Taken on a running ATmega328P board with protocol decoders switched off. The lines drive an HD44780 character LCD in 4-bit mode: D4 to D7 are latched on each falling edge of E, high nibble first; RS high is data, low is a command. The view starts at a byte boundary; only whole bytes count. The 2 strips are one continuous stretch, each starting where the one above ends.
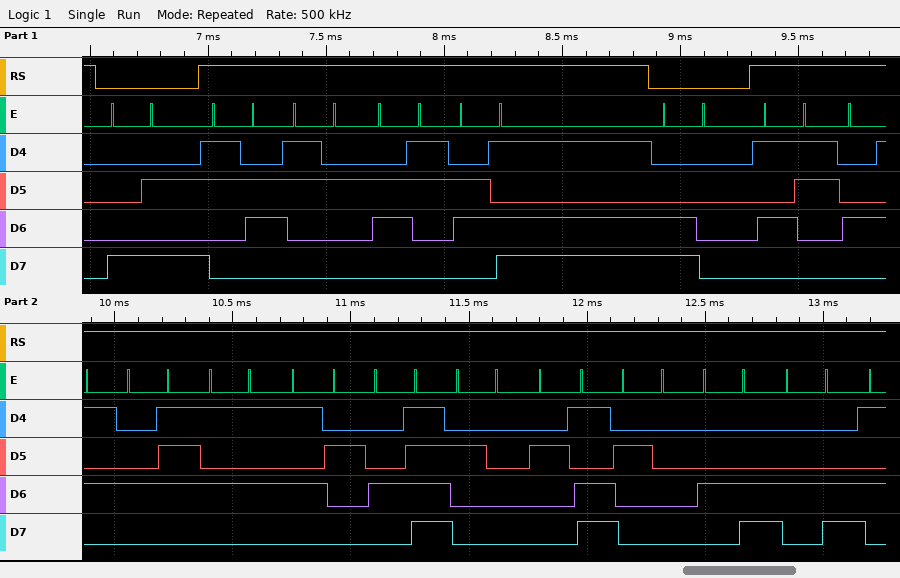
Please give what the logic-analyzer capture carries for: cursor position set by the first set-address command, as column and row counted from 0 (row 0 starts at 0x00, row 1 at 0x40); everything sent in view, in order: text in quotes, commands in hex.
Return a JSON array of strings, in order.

["column 10, row 0", "0x8A \"62cm\" 0xC0 \"SEGURO - LL\""]
